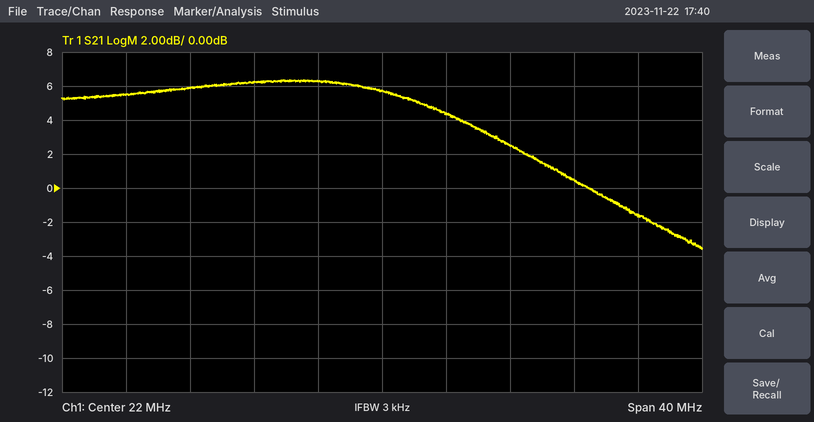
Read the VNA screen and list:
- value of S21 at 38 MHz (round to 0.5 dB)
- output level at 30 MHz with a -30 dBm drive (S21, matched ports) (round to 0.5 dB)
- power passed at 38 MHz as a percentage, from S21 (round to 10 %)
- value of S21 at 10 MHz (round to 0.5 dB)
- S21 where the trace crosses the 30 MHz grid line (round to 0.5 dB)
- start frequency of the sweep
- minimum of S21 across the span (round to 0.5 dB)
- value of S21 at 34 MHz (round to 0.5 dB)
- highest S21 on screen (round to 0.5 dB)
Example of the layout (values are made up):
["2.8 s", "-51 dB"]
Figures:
["-1.5 dB", "-27.5 dBm", "70 %", "6.0 dB", "2.5 dB", "2 MHz", "-3.5 dB", "0.5 dB", "6.5 dB"]
